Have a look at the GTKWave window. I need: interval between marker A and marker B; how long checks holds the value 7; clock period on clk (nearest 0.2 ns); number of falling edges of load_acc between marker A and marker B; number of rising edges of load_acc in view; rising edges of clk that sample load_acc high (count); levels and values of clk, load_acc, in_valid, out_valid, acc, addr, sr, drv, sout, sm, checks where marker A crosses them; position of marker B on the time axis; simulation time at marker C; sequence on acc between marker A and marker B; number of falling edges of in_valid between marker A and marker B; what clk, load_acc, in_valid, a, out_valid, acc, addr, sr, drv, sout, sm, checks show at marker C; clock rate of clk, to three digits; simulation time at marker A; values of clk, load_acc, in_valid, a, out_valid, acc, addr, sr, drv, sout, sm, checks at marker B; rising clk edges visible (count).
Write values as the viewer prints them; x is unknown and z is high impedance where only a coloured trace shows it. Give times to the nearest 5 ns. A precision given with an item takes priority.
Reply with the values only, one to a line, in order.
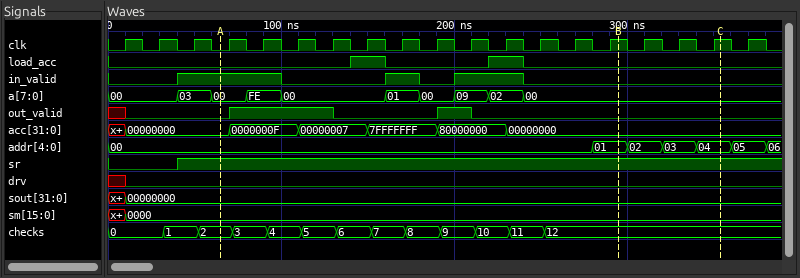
230 ns
20 ns
20 ns
2
2
2
clk=0, load_acc=0, in_valid=1, out_valid=0, acc=00000000, addr=00, sr=1, drv=0, sout=00000000, sm=0000, checks=2
295 ns
355 ns
00000000, 0000000F, 00000007, 7FFFFFFF, 80000000, 00000000
3
clk=1, load_acc=0, in_valid=0, a=00, out_valid=0, acc=00000000, addr=04, sr=1, drv=0, sout=00000000, sm=0000, checks=12
50.0 MHz
65 ns
clk=1, load_acc=0, in_valid=0, a=00, out_valid=0, acc=00000000, addr=01, sr=1, drv=0, sout=00000000, sm=0000, checks=12
19
